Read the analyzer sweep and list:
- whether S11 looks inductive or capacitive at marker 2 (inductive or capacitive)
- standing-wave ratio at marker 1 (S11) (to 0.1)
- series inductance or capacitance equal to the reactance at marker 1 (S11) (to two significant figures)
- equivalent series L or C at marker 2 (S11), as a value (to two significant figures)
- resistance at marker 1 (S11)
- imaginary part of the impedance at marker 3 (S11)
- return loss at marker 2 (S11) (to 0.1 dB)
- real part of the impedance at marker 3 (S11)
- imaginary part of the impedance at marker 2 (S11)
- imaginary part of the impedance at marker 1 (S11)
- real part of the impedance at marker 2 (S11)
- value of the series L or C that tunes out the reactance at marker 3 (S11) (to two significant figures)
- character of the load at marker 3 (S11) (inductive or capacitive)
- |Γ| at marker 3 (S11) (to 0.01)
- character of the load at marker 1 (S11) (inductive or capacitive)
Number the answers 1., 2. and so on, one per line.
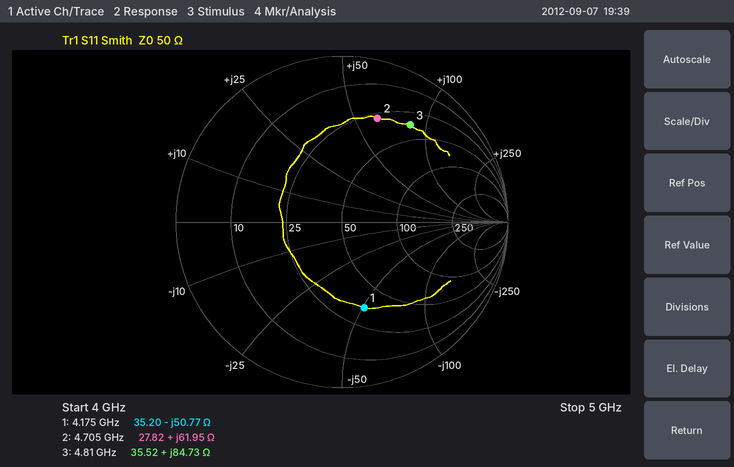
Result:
1. inductive
2. 3.3
3. 750 fF
4. 2.1 nH
5. 35.20 Ω
6. +84.73 Ω
7. 3.6 dB
8. 35.52 Ω
9. +61.95 Ω
10. -50.77 Ω
11. 27.82 Ω
12. 390 fF
13. inductive
14. 0.71
15. capacitive
